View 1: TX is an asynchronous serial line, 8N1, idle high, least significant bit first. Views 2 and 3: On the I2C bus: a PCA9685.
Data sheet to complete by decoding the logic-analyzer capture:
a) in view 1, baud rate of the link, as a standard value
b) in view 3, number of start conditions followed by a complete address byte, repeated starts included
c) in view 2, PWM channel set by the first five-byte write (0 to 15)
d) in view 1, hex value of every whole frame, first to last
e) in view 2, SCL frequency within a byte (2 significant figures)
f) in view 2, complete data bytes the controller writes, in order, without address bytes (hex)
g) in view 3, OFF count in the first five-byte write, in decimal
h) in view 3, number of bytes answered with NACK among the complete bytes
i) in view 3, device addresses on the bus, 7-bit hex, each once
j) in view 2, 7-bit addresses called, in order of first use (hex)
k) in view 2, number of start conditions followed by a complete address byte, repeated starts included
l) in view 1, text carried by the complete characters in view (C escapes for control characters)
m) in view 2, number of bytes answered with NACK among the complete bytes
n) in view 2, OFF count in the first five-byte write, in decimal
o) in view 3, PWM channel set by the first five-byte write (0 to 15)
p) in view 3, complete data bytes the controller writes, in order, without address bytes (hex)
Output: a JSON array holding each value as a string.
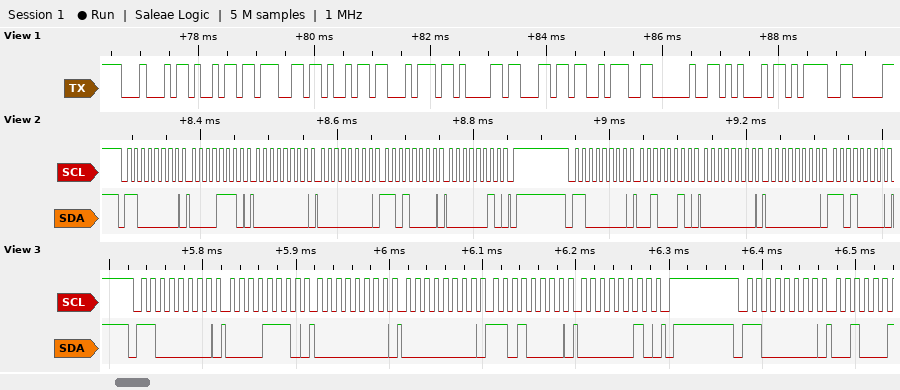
["9600 baud", "2", "2", "44 69 67 69 74 61 6C 3A 20 45 3D", "100 kHz", "0E 00 00 D0 02 22 00 00 D0", "720", "0", "0x60", "0x60", "2", "\"Digital: E=\"", "0", "720", "2", "0E 00 00 D0 02"]
